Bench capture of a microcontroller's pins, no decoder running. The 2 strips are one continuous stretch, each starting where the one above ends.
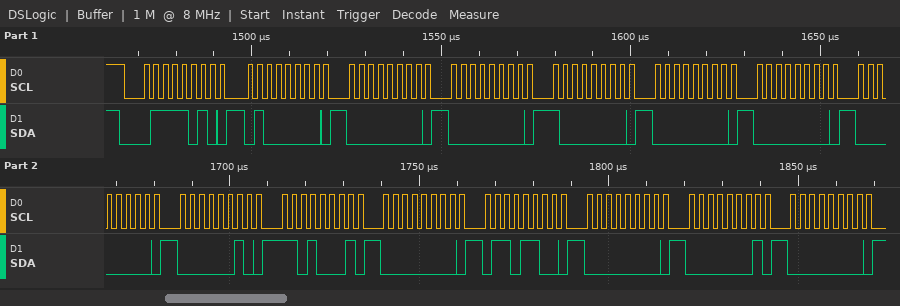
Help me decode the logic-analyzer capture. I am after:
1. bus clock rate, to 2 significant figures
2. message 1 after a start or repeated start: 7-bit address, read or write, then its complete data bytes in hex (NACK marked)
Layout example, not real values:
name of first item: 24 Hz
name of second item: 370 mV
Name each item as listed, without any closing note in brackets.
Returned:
bus clock rate, to 2 significant figures: 400 kHz
message 1 after a start or repeated start: 7-bit address, read or write, then its complete data bytes in hex: 0x3D write: 40 00 00 80 00 00 00 02 D1 00 6C 00 01 00
